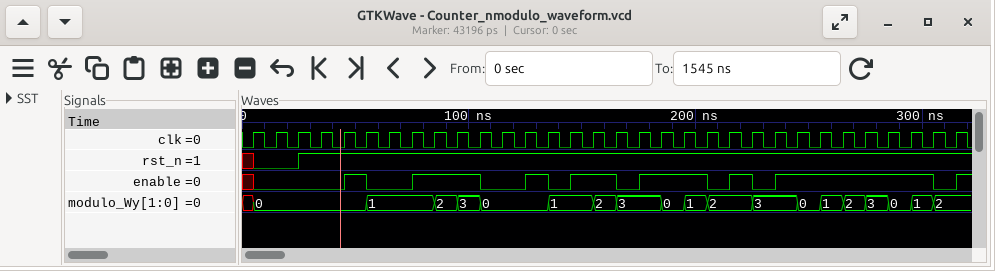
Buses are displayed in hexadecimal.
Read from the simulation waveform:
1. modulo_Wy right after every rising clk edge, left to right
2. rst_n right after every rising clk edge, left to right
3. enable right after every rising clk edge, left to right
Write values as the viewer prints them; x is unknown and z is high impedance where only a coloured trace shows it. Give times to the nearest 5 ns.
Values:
0, 0, 0, 0, 0, 1, 1, 1, 2, 3, 0, 0, 0, 1, 1, 2, 3, 3, 0, 1, 2, 2, 3, 3, 0, 1, 2, 3, 0, 1, 2, 2
0 0 1 1 1 1 1 1 1 1 1 1 1 1 1 1 1 1 1 1 1 1 1 1 1 1 1 1 1 1 1 1
0 0 0 0 1 0 0 1 1 1 0 0 1 0 1 1 0 1 1 1 0 1 0 1 1 1 1 1 1 1 0 1
